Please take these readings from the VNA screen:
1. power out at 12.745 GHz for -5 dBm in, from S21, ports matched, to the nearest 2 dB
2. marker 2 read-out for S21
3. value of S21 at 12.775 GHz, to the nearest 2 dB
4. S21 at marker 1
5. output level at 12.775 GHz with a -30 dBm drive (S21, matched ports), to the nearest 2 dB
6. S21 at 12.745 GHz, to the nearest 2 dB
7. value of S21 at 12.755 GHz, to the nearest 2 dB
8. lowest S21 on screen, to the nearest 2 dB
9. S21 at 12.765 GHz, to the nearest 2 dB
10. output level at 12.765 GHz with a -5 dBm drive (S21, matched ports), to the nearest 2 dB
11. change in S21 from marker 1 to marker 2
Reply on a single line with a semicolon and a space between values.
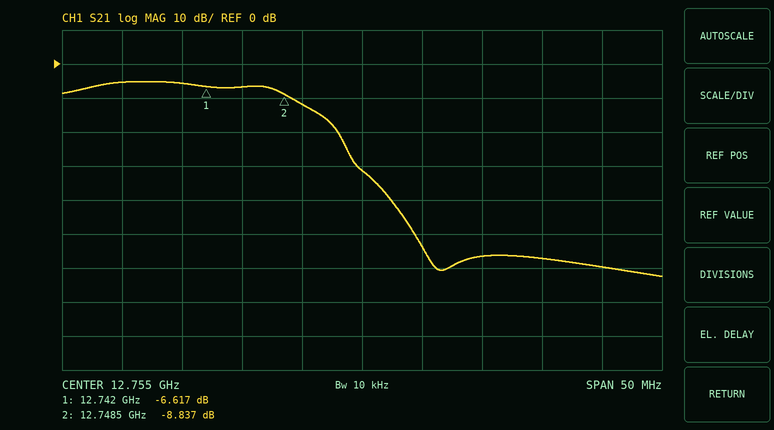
-12 dBm; -8.837 dB; -60 dB; -6.617 dB; -90 dBm; -6 dB; -32 dB; -62 dB; -56 dB; -62 dBm; -2.220 dB
